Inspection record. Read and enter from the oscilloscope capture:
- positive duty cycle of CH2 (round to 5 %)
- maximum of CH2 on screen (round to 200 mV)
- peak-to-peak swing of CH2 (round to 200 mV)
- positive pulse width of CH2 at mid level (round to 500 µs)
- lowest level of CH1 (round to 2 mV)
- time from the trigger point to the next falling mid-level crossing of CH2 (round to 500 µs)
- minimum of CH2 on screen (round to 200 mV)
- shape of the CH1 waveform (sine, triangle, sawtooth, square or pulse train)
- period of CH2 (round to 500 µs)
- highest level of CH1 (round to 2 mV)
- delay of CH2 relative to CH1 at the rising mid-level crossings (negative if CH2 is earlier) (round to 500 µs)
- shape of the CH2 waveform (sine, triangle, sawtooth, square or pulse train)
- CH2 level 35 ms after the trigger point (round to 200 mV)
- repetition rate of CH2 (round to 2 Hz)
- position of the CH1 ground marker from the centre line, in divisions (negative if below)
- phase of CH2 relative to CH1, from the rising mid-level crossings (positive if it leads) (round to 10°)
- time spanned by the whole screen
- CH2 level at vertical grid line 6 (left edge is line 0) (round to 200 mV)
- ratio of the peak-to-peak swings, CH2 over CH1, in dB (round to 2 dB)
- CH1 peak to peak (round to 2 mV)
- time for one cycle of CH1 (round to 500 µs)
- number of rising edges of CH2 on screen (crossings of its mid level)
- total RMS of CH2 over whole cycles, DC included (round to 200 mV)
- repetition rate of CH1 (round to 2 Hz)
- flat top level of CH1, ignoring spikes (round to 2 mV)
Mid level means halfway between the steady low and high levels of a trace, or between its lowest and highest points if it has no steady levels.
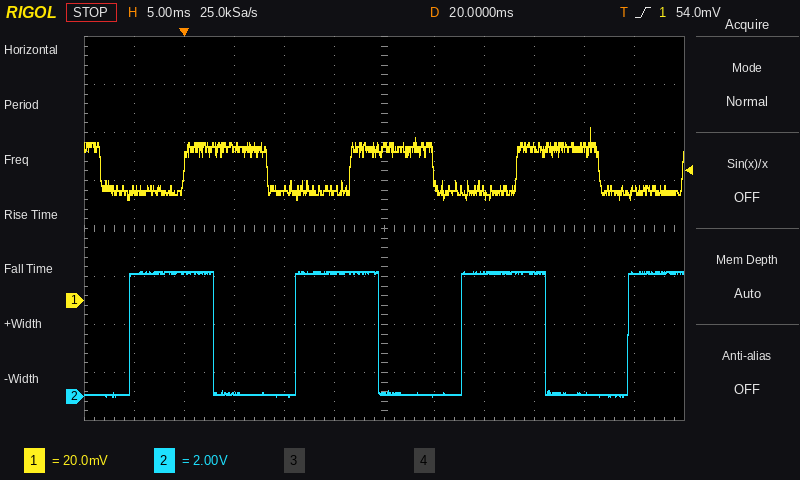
50 %
5.2 V
5.2 V
8.5 ms
42 mV
3.0 ms
0.0 V
square
16.5 ms
72 mV
-5.5 ms
square
5.2 V
60 Hz
-1.5 div
+120°
60 ms
200 mV
44 dB
30 mV
16.5 ms
4
3.6 V
60 Hz
64 mV
